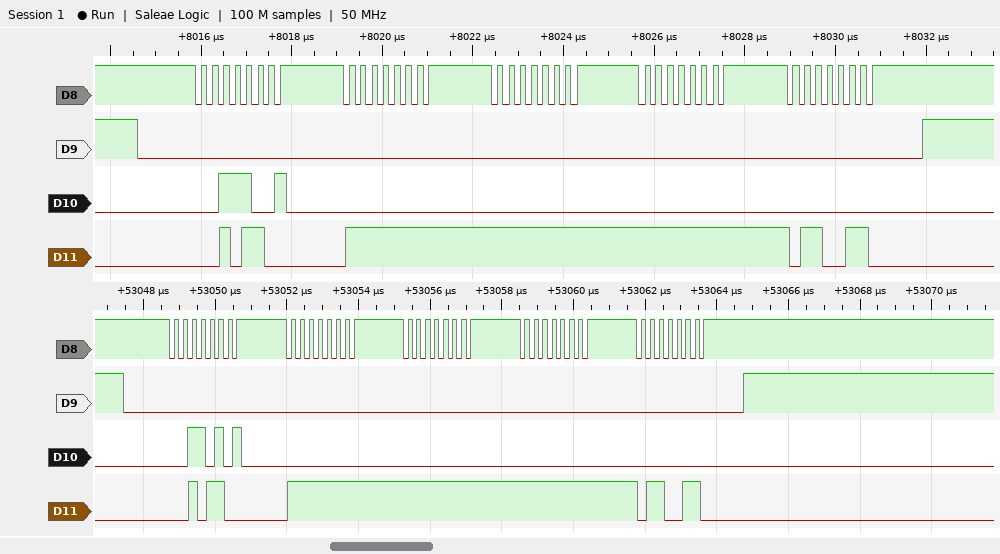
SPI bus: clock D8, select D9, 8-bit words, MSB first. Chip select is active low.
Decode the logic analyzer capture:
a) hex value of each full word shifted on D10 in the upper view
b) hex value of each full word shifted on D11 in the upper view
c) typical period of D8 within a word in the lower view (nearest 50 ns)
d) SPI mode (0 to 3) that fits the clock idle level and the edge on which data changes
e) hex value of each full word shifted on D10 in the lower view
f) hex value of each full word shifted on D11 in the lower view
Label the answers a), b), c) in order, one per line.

a) 39, 00, 00, 00, 00
b) 2C, FF, FF, FF, 66
c) 250 ns
d) 3
e) 35, 00, 00, 00, 00
f) 2C, FF, FF, FF, 66
